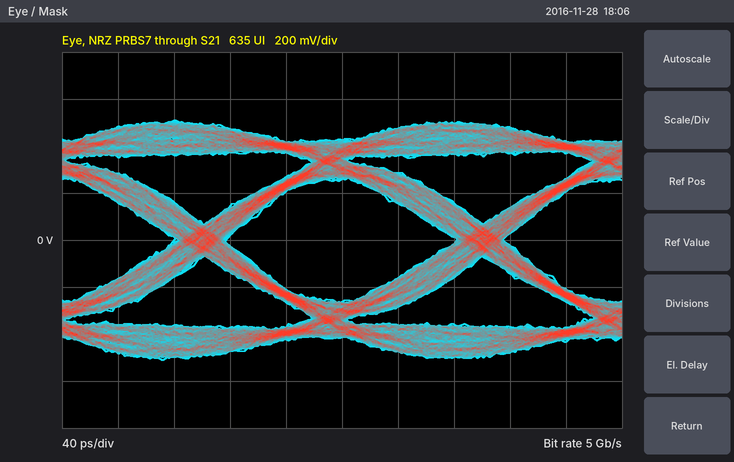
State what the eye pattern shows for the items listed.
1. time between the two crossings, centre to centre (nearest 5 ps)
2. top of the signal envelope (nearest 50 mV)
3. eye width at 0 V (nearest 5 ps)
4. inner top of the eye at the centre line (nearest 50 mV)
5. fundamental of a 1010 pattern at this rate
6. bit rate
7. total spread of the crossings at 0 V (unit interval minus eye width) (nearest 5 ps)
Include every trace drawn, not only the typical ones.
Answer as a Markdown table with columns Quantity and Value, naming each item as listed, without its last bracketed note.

| Quantity | Value |
|---|---|
| time between the two crossings, centre to centre | 200 ps |
| top of the signal envelope | 500 mV |
| eye width at 0 V | 165 ps |
| inner top of the eye at the centre line | 250 mV |
| fundamental of a 1010 pattern at this rate | 2.5 GHz |
| bit rate | 5 Gb/s |
| total spread of the crossings at 0 V (unit interval minus eye width) | 35 ps |
